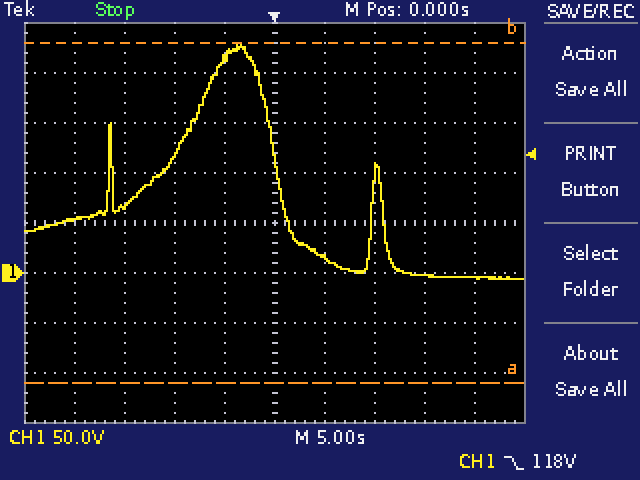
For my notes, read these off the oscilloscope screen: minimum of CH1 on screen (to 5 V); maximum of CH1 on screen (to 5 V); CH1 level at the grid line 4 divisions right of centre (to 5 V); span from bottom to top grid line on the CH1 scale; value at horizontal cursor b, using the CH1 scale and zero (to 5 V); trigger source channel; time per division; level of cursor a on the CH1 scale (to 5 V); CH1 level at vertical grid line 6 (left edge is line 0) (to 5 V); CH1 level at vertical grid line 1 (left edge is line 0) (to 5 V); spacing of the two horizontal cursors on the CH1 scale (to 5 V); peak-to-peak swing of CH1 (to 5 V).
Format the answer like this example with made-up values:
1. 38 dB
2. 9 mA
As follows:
1. -5 V
2. 230 V
3. -5 V
4. 400 V
5. 230 V
6. CH1
7. 5 s
8. -110 V
9. 15 V
10. 55 V
11. 340 V
12. 235 V
